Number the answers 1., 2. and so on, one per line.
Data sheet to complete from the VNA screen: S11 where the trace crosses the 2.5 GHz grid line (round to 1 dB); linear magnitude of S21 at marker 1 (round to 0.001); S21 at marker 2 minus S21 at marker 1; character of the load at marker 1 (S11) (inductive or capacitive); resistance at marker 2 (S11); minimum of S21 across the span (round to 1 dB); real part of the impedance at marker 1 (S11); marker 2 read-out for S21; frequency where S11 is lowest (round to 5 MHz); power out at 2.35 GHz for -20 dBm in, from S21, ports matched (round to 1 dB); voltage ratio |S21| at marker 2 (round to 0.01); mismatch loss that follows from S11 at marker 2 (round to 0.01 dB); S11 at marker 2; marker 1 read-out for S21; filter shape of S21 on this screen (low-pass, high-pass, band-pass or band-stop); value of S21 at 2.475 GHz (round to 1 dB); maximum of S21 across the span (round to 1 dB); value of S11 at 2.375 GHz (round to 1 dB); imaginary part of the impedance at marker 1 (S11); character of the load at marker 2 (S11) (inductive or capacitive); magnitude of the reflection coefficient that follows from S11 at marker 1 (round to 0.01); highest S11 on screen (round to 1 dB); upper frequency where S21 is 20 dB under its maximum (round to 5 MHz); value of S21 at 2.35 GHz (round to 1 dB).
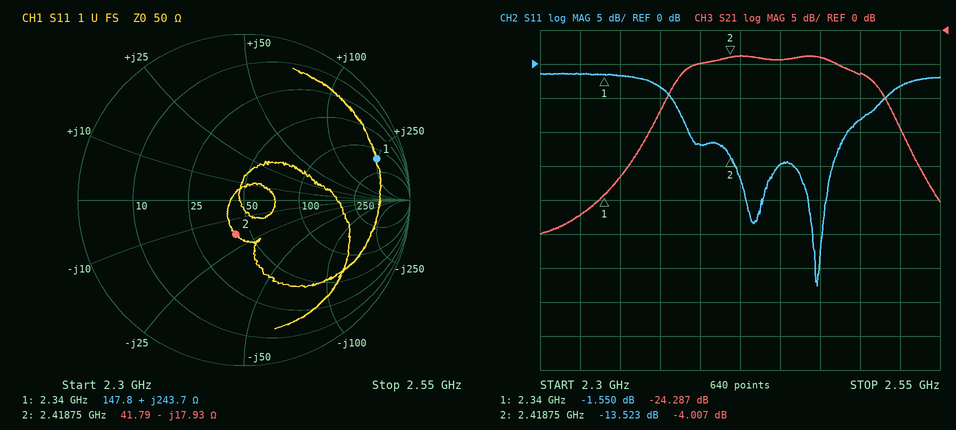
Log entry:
1. -8 dB
2. 0.061
3. 20.280 dB
4. inductive
5. 41.79 Ω
6. -30 dB
7. 147.8 Ω
8. -4.007 dB
9. 2.475 GHz
10. -42 dBm
11. 0.63
12. 0.20 dB
13. -13.523 dB
14. -24.287 dB
15. band-pass
16. -4 dB
17. -4 dB
18. -3 dB
19. +243.7 Ω
20. capacitive
21. 0.84
22. -1 dB
23. 2.545 GHz
24. -22 dB
